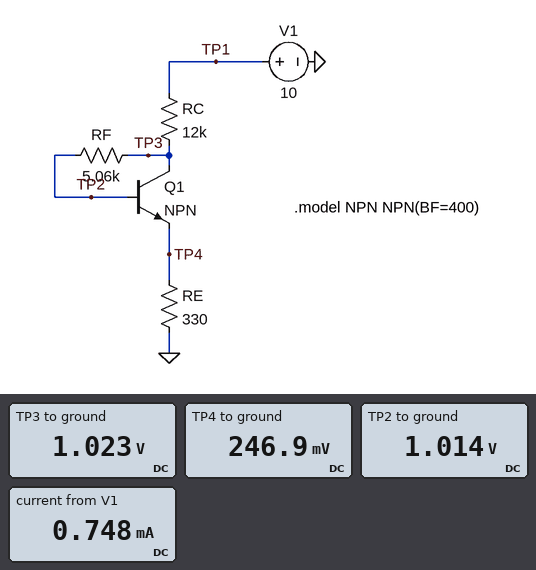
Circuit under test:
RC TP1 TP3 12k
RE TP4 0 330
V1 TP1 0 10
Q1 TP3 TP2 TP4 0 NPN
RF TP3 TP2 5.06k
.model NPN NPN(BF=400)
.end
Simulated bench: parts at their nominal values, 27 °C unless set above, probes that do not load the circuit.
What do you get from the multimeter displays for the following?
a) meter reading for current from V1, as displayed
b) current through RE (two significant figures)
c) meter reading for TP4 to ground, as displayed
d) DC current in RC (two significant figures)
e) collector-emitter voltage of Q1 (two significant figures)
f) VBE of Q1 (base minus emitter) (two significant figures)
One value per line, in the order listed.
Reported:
0.748 mA
750 µA
246.9 mV
750 µA
780 mV
770 mV
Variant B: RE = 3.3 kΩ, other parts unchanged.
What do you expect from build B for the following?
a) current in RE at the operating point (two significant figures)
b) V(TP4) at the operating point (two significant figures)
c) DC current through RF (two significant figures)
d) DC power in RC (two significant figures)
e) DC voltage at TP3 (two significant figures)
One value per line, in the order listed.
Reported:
600 µA
2.0 V
1.5 µA
4.4 mW
2.8 V
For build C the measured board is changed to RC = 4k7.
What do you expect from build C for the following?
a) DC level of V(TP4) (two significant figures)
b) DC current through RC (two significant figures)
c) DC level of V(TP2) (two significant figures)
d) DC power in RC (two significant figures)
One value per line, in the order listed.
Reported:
600 mV
1.8 mA
1.4 V
16 mW
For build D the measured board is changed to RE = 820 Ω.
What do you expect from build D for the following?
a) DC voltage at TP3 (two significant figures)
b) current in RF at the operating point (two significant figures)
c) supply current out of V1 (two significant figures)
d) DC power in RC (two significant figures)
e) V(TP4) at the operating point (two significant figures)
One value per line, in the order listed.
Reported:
1.4 V
1.8 µA
720 µA
6.2 mW
590 mV
